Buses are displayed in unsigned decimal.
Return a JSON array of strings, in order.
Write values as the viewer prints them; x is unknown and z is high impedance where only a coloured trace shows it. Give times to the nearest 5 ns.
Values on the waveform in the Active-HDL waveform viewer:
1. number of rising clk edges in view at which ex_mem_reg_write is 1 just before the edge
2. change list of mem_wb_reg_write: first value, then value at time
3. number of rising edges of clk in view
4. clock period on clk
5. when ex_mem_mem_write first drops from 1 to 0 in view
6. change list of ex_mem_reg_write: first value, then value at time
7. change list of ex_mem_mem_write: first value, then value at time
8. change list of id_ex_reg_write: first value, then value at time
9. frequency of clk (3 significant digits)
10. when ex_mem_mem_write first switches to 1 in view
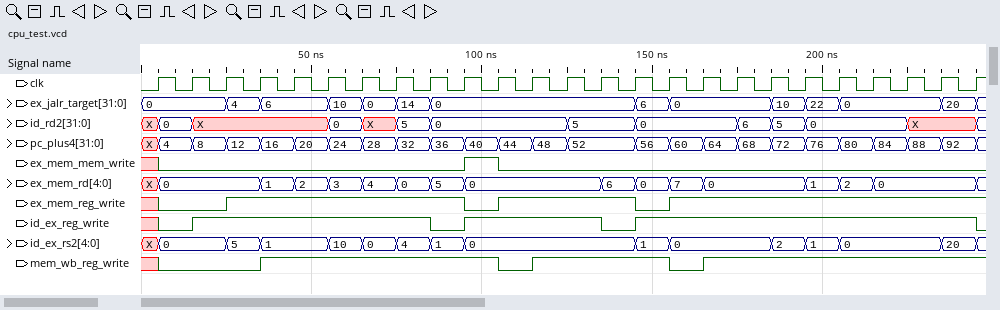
["20", "x, 0 at 5 ns, 1 at 35 ns, 0 at 105 ns, 1 at 115 ns, 0 at 155 ns, 1 at 165 ns", "25", "10 ns", "105 ns", "x, 0 at 5 ns, 1 at 25 ns, 0 at 95 ns, 1 at 105 ns, 0 at 145 ns, 1 at 155 ns", "x, 0 at 5 ns, 1 at 95 ns, 0 at 105 ns", "x, 0 at 5 ns, 1 at 15 ns, 0 at 85 ns, 1 at 95 ns, 0 at 135 ns, 1 at 145 ns, 0 at 245 ns", "100 MHz", "95 ns"]
